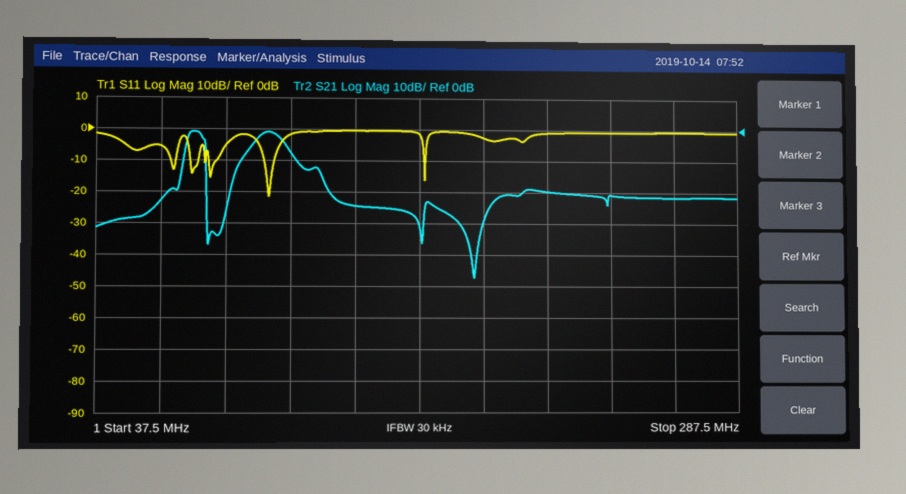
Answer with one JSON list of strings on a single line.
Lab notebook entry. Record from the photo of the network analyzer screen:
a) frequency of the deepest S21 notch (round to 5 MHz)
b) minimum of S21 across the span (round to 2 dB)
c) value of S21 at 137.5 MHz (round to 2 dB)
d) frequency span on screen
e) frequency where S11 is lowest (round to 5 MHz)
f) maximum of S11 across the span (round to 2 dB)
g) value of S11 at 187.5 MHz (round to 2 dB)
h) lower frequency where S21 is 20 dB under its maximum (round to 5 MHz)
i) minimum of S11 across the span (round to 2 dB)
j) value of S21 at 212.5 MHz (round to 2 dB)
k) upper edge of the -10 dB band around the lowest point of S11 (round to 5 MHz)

["185 MHz", "-48 dB", "-24 dB", "250 MHz", "105 MHz", "0 dB", "-2 dB", "65 MHz", "-22 dB", "-20 dB", "105 MHz"]
